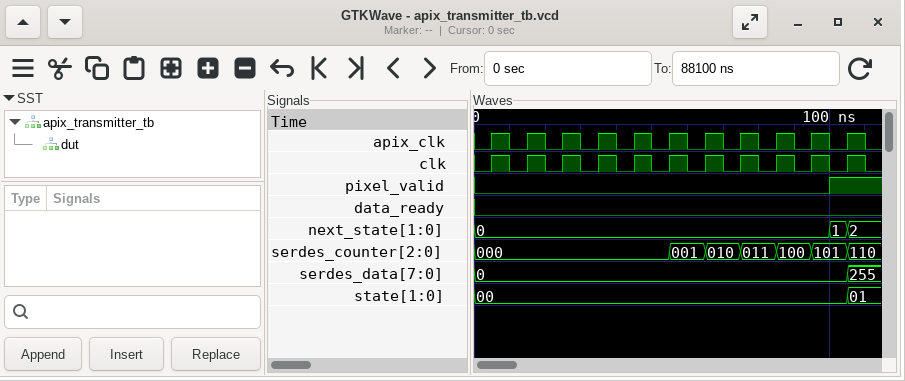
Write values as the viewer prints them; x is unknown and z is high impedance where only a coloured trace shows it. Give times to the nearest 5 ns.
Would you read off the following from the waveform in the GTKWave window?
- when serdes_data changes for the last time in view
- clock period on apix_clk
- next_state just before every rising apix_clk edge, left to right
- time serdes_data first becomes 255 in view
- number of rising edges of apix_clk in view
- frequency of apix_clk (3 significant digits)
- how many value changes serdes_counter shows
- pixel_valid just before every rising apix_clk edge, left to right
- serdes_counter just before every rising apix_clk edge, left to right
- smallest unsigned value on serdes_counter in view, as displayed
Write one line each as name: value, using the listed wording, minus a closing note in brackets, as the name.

when serdes_data changes for the last time in view: 105 ns
clock period on apix_clk: 10 ns
next_state just before every rising apix_clk edge, left to right: 0, 0, 0, 0, 0, 0, 0, 0, 0, 0, 1
time serdes_data first becomes 255 in view: 105 ns
number of rising edges of apix_clk in view: 11
frequency of apix_clk: 100 MHz
how many value changes serdes_counter shows: 6
pixel_valid just before every rising apix_clk edge, left to right: 0 0 0 0 0 0 0 0 0 0 1
serdes_counter just before every rising apix_clk edge, left to right: 000, 000, 000, 000, 000, 000, 001, 010, 011, 100, 101
smallest unsigned value on serdes_counter in view, as displayed: 000
